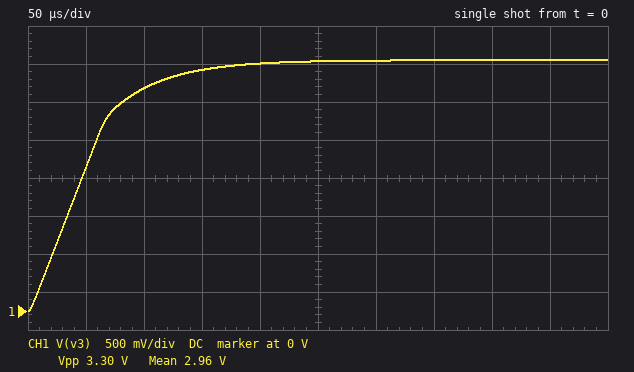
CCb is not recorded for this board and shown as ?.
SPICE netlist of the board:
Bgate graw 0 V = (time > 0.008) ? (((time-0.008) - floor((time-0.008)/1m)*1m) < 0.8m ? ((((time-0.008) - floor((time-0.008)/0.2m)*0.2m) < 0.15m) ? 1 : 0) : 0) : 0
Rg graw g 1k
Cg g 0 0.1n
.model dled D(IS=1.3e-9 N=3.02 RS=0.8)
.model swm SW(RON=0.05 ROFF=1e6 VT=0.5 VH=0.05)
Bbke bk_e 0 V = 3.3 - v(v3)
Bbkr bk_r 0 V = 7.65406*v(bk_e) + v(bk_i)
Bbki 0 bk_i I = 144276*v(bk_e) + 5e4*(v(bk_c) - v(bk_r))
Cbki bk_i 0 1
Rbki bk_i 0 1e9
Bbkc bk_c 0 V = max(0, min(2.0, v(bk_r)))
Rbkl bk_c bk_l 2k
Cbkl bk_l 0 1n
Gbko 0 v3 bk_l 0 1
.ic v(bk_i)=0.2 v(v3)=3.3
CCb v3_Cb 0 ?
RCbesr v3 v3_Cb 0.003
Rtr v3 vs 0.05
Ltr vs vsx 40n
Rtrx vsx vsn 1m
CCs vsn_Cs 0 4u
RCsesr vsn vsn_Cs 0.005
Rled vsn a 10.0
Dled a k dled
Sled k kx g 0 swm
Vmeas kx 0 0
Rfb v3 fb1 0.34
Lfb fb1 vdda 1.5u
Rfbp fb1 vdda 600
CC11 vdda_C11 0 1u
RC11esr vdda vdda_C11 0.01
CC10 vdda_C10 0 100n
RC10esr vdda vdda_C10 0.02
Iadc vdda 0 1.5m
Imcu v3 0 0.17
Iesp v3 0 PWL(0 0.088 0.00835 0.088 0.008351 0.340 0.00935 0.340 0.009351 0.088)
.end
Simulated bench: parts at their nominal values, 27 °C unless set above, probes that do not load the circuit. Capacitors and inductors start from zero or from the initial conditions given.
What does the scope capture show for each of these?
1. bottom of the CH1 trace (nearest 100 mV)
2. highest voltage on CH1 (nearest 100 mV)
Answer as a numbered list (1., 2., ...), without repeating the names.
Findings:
1. 0 V
2. 3.3 V
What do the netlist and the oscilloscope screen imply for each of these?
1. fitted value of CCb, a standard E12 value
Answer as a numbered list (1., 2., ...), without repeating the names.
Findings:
1. 39 µF
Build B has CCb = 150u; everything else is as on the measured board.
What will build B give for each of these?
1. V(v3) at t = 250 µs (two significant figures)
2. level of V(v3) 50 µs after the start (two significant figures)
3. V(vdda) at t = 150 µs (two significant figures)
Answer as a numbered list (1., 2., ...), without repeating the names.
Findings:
1. 2.8 V
2. 540 mV
3. 1.7 V
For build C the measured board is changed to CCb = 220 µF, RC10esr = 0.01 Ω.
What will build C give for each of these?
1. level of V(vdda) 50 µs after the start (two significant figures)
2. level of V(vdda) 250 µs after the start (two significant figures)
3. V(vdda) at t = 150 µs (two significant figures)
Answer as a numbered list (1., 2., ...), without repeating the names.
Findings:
1. 370 mV
2. 1.9 V
3. 1.1 V
